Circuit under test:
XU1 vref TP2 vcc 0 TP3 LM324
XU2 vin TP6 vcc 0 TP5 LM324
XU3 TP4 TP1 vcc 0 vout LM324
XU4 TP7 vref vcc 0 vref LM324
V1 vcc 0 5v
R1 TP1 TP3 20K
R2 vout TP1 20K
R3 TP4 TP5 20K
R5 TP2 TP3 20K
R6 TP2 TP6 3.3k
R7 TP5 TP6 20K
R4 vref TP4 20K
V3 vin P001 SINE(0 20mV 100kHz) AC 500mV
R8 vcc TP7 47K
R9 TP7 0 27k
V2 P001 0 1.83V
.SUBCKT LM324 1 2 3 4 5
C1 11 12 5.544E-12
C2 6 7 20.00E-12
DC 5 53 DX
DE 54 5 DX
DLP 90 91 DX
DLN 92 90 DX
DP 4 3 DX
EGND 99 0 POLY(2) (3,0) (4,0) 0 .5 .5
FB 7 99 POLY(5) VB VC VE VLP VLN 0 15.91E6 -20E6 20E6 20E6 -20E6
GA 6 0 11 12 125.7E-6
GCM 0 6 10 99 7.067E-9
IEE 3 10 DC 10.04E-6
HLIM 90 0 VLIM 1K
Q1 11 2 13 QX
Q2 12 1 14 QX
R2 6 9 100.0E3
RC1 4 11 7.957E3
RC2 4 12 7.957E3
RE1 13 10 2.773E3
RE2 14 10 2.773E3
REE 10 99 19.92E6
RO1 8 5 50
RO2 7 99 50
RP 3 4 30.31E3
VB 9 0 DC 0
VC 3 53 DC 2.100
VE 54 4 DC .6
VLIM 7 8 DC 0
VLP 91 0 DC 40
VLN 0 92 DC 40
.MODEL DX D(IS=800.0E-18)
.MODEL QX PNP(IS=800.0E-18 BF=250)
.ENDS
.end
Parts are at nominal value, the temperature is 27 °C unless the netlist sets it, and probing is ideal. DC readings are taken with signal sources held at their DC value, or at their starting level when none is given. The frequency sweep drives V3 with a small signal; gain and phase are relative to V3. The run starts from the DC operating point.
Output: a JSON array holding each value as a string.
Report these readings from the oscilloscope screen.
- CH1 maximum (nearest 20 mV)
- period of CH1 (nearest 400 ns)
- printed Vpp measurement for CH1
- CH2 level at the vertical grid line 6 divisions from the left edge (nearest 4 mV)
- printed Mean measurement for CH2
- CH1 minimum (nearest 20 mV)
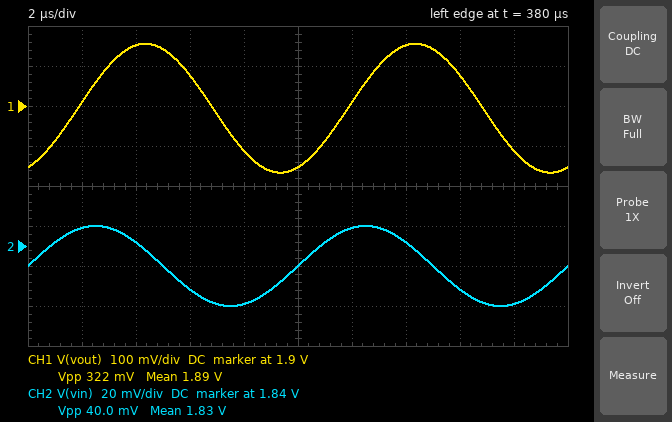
["2.06 V", "10.0 µs", "322 mV", "1.848 V", "1.83 V", "1.74 V"]
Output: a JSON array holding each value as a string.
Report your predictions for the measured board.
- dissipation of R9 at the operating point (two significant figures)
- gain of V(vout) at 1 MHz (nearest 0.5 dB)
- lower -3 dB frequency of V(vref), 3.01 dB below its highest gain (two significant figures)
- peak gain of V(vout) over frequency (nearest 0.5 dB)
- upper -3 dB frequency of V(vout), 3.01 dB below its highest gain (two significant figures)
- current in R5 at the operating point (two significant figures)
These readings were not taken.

["120 µW", "-7.0 dB", "380 kHz", "22.5 dB", "78 kHz", "1.6 µA"]
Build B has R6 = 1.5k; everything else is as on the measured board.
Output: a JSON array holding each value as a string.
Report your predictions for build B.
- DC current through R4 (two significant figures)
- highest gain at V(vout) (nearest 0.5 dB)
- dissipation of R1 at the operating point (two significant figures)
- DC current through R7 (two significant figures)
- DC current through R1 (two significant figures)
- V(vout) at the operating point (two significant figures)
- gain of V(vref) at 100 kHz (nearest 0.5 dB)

["1.9 µA", "29.0 dB", "600 nW", "3.5 µA", "5.5 µA", "2.0 V", "-64.0 dB"]
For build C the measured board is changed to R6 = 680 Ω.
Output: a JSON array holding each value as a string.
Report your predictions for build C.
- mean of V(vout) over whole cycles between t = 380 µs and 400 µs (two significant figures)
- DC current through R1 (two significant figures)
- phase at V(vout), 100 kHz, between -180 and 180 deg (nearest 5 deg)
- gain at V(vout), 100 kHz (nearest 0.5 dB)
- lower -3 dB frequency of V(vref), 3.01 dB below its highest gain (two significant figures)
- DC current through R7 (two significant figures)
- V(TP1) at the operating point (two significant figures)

["2.1 V", "12 µA", "-95 deg", "20.0 dB", "430 kHz", "7.8 µA", "1.9 V"]
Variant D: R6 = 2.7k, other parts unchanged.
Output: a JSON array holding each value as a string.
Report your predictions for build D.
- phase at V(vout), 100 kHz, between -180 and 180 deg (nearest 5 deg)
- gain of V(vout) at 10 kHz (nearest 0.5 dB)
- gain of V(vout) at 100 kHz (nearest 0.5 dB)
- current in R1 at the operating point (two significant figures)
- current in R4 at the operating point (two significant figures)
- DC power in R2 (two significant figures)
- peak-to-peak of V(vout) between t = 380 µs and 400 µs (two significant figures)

["-70 deg", "24.0 dB", "18.5 dB", "3.1 µA", "1.1 µA", "190 nW", "340 mV"]
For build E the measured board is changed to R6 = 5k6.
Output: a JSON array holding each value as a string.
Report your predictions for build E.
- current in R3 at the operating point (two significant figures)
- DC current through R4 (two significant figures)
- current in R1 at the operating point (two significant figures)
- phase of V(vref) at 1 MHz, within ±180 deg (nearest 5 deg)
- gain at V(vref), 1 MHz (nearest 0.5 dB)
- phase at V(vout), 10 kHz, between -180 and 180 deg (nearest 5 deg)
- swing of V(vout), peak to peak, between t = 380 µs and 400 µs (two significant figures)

["590 nA", "610 nA", "1.6 µA", "-35 deg", "-59.0 dB", "-5 deg", "260 mV"]
